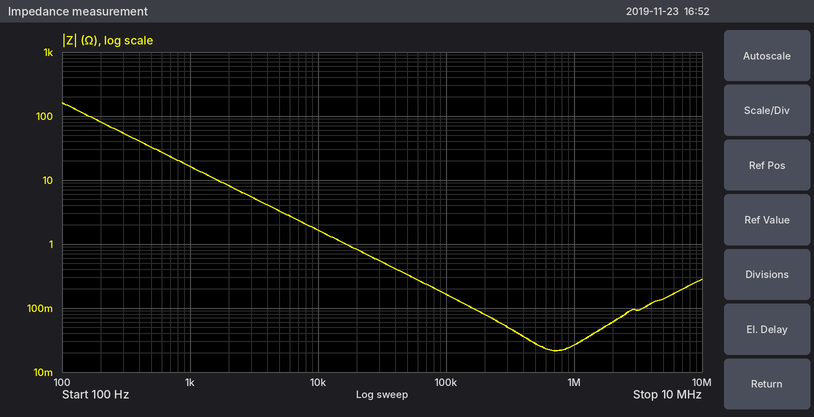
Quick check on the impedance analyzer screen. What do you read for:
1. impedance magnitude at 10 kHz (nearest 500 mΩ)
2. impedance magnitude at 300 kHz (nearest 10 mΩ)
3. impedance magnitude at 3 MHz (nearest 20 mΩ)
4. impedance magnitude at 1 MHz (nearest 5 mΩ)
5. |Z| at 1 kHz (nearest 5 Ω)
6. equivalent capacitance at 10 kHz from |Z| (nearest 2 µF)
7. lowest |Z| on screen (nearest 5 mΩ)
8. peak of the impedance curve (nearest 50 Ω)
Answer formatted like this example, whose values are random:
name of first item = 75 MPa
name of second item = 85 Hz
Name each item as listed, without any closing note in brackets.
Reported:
impedance magnitude at 10 kHz = 1.5 Ω
impedance magnitude at 300 kHz = 50 mΩ
impedance magnitude at 3 MHz = 100 mΩ
impedance magnitude at 1 MHz = 25 mΩ
|Z| at 1 kHz = 15 Ω
equivalent capacitance at 10 kHz from |Z| = 10 µF
lowest |Z| on screen = 20 mΩ
peak of the impedance curve = 150 Ω
